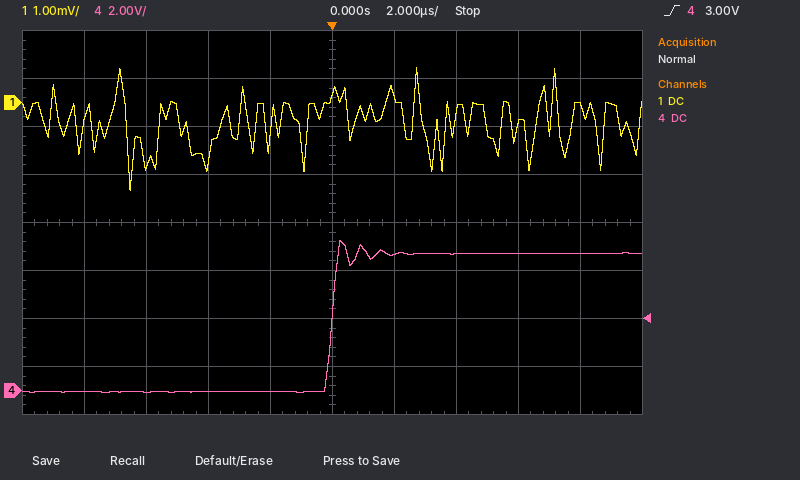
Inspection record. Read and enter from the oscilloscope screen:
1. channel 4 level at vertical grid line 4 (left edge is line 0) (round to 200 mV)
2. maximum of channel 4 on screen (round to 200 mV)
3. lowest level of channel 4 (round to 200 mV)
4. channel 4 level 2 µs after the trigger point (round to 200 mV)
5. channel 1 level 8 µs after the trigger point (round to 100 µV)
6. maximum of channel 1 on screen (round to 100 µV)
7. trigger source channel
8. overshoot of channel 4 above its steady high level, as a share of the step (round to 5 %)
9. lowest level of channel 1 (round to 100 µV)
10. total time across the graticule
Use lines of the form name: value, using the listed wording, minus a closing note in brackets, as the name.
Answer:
channel 4 level at vertical grid line 4 (left edge is line 0): 0.0 V
maximum of channel 4 on screen: 6.2 V
lowest level of channel 4: 0.0 V
channel 4 level 2 µs after the trigger point: 5.6 V
channel 1 level 8 µs after the trigger point: -100 µV
maximum of channel 1 on screen: 700 µV
trigger source channel: channel 4
overshoot of channel 4 above its steady high level, as a share of the step: 10 %
lowest level of channel 1: -1.8 mV
total time across the graticule: 20 µs
